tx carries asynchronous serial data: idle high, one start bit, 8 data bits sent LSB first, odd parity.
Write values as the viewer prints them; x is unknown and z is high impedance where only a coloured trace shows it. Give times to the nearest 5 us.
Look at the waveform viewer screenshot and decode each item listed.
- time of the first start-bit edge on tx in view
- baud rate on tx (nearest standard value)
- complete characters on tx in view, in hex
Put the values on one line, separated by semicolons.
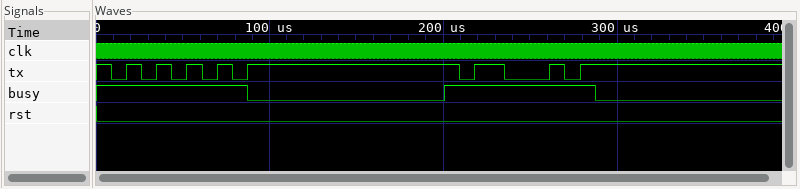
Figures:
10 us; 115200 baud; 55, A3
